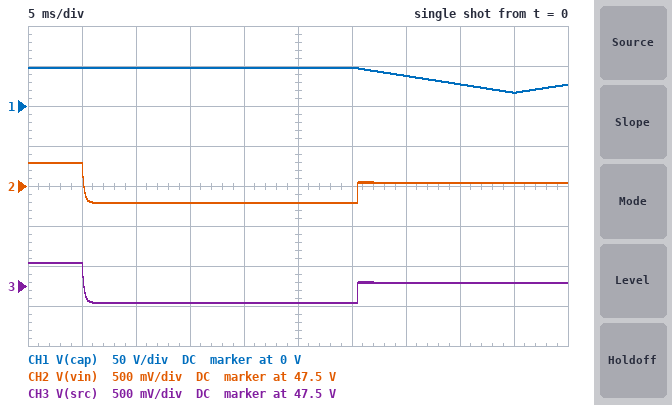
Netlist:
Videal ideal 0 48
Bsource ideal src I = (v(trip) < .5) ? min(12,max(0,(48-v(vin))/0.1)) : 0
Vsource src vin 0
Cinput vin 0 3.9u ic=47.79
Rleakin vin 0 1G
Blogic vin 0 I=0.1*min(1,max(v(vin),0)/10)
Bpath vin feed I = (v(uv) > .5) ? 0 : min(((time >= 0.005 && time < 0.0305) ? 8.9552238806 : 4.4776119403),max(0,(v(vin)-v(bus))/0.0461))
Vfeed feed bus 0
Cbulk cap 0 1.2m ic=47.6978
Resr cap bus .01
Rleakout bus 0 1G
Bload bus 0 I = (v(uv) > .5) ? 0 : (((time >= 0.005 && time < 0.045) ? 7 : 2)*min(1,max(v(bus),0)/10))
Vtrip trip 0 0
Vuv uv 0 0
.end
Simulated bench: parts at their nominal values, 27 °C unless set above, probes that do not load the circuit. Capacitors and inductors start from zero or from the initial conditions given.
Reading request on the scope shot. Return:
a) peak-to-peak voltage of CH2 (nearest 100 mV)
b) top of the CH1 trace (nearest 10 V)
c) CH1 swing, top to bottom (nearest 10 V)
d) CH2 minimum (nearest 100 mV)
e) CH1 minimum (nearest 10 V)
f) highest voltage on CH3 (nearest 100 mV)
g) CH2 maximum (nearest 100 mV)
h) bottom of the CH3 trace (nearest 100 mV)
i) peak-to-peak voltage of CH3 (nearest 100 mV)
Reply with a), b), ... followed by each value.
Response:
a) 500 mV
b) 50 V
c) 30 V
d) 47.3 V
e) 20 V
f) 47.8 V
g) 47.8 V
h) 47.3 V
i) 500 mV
